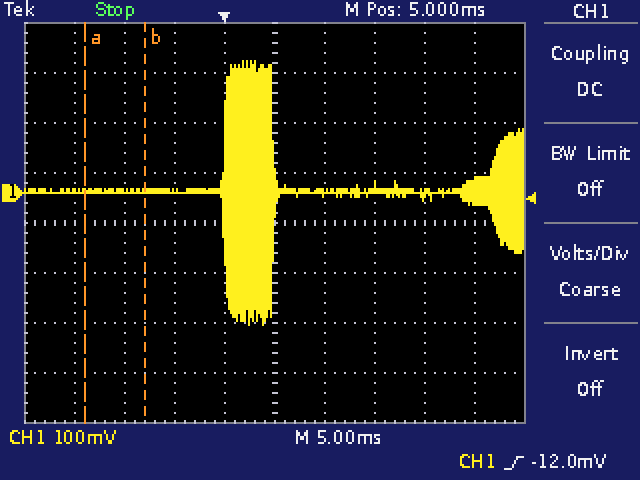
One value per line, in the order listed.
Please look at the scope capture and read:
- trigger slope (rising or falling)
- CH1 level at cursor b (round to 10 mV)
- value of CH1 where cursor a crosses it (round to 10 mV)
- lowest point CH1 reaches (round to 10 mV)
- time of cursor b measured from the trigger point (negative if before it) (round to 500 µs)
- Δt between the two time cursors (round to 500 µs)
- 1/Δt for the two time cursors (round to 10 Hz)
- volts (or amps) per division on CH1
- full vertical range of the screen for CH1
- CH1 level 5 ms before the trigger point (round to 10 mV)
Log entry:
rising
0 mV
0 mV
-260 mV
-8.0 ms
6.0 ms
170 Hz
100 mV
800 mV
0 mV
